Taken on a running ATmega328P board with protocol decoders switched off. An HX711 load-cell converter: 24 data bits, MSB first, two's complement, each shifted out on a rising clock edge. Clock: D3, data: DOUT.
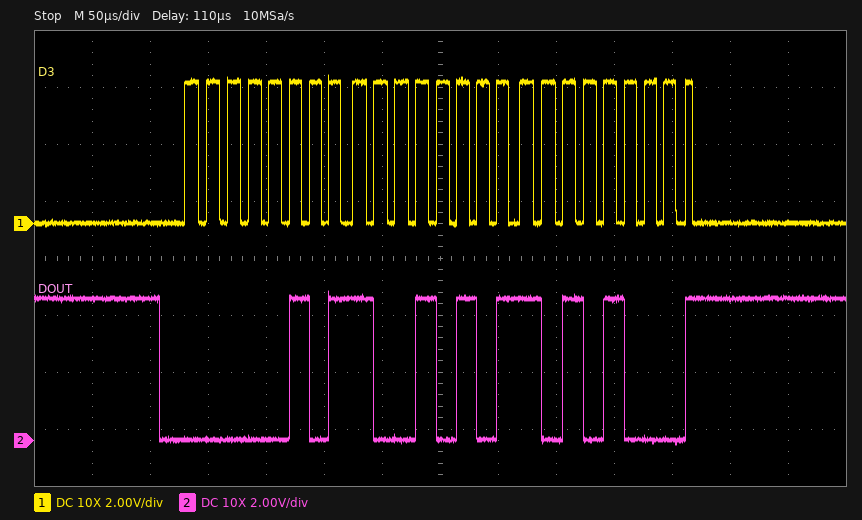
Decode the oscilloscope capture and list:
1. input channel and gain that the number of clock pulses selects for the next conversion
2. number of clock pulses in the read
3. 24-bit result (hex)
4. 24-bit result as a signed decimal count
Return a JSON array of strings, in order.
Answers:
["channel A, gain 128", "25", "0x0595A8", "365992"]
